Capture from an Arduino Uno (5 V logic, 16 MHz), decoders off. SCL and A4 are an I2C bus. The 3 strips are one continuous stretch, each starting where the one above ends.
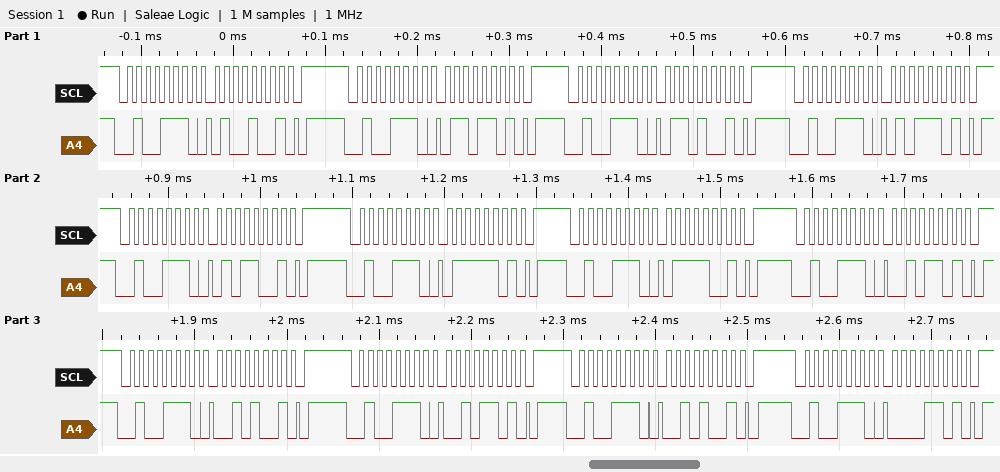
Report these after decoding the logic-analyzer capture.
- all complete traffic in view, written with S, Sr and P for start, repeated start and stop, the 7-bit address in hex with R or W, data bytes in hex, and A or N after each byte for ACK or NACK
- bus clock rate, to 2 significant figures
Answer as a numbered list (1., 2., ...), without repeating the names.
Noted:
1. S 27W A 49 A P S 27W A 6D A P S 27W A 69 A P S 27W A 5D A P S 27W A 59 A P S 27W A 7D A P S 27W A 79 A P S 27W A 2D A P S 27W A 29 A P S 27W A 2D A P S 27W A 29 A P S 27W A 0D A P
2. 100 kHz
